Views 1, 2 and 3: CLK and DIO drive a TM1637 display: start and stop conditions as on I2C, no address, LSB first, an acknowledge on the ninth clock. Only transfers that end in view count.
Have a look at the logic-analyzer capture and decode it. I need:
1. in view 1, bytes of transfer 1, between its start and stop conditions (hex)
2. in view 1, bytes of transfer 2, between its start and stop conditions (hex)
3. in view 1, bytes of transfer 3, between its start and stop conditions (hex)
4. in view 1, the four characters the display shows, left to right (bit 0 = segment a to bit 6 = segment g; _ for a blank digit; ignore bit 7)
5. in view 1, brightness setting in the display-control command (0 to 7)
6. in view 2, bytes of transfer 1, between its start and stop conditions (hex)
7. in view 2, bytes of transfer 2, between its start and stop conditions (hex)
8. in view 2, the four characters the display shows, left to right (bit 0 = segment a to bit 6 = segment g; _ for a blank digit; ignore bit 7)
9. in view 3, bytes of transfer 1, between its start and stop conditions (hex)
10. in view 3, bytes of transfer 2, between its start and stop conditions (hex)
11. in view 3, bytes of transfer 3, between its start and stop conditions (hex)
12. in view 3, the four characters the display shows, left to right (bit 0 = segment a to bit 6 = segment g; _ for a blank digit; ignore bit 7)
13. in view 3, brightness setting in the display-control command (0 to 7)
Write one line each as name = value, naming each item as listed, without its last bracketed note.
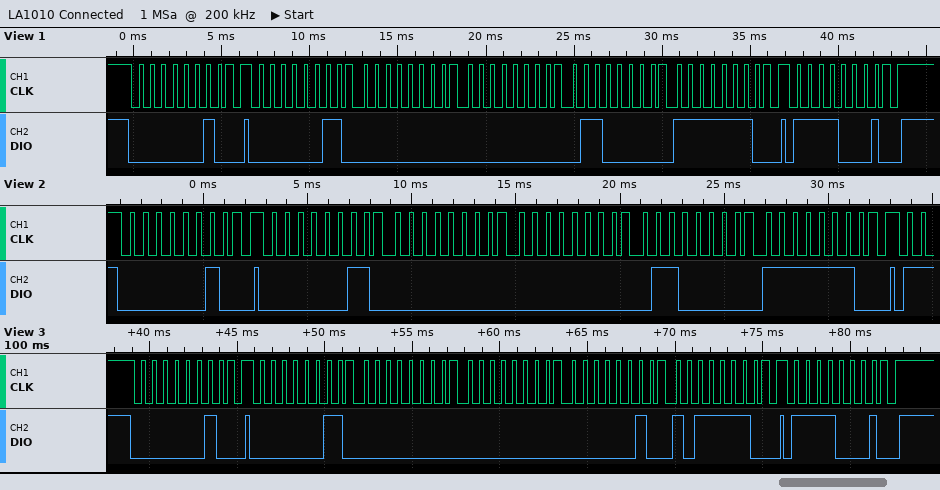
in view 1, bytes of transfer 1, between its start and stop conditions = 40
in view 1, bytes of transfer 2, between its start and stop conditions = C0 00 00 06 7F
in view 1, bytes of transfer 3, between its start and stop conditions = 8F
in view 1, the four characters the display shows, left to right = __18
in view 1, brightness setting in the display-control command = 7
in view 2, bytes of transfer 1, between its start and stop conditions = 40
in view 2, bytes of transfer 2, between its start and stop conditions = C0 00 00 06 7F
in view 2, the four characters the display shows, left to right = __18
in view 3, bytes of transfer 1, between its start and stop conditions = 40
in view 3, bytes of transfer 2, between its start and stop conditions = C0 00 00 40 7D
in view 3, bytes of transfer 3, between its start and stop conditions = 8F
in view 3, the four characters the display shows, left to right = __-6
in view 3, brightness setting in the display-control command = 7
